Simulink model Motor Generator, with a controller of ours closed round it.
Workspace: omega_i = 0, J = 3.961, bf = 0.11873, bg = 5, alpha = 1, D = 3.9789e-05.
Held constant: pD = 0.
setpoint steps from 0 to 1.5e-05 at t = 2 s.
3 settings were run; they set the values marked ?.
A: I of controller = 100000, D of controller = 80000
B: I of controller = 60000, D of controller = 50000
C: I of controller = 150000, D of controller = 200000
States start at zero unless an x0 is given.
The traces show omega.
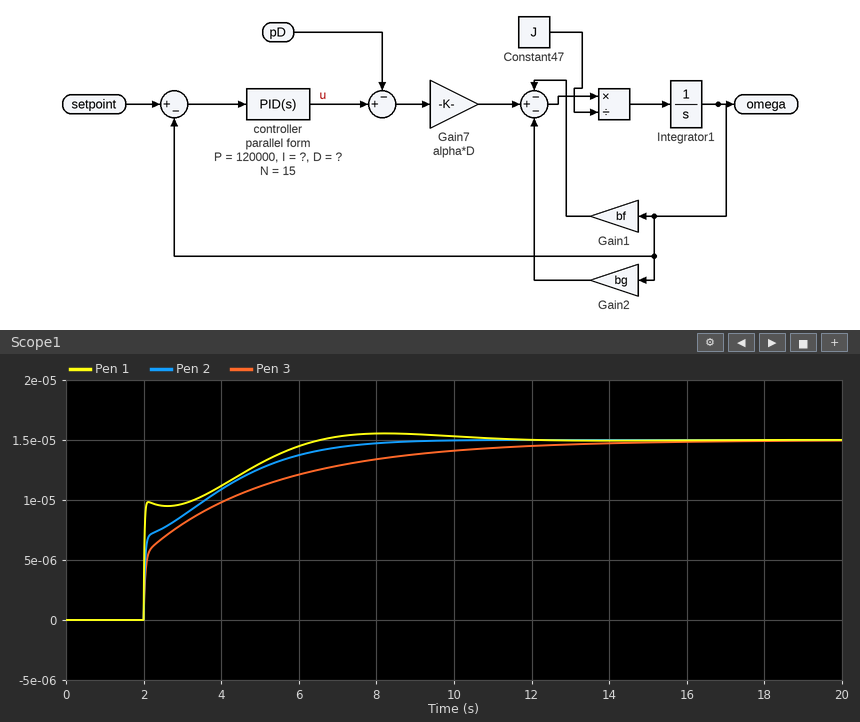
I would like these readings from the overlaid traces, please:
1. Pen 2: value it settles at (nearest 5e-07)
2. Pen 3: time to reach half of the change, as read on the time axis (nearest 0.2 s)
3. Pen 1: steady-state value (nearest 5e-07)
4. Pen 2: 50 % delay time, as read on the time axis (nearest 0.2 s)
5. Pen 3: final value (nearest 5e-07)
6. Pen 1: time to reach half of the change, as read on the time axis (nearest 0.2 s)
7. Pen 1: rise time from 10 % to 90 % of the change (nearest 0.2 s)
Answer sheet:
0.0000150
2.8 s
0.0000150
2.4 s
0.0000150
2.0 s
3.2 s
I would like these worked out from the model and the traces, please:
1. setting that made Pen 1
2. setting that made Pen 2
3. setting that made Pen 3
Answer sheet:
C
A
B
